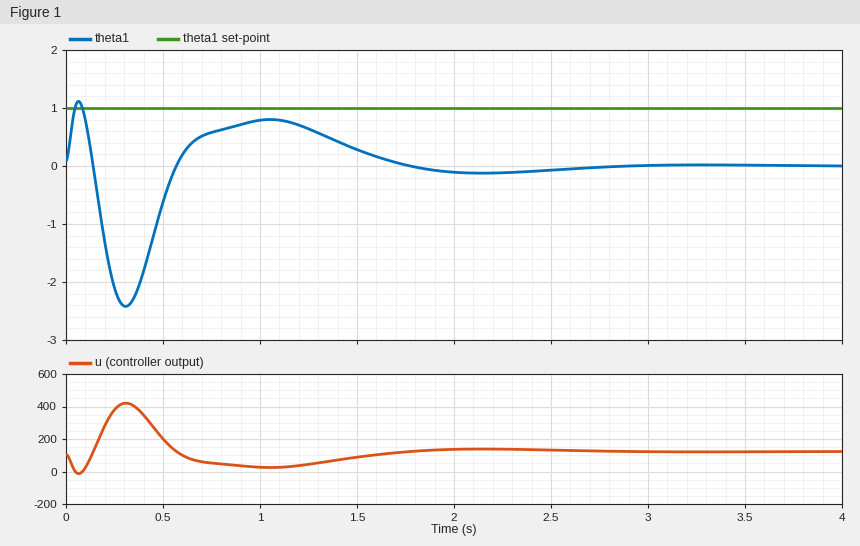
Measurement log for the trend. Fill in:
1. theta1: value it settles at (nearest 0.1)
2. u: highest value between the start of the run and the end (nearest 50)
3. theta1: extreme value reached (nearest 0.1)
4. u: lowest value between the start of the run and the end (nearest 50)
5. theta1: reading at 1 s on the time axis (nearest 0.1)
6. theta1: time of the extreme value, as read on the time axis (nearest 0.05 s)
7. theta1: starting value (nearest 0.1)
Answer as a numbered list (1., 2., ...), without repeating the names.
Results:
1. 0.0
2. 400
3. -2.4
4. 0
5. 0.8
6. 0.30 s
7. 0.1
